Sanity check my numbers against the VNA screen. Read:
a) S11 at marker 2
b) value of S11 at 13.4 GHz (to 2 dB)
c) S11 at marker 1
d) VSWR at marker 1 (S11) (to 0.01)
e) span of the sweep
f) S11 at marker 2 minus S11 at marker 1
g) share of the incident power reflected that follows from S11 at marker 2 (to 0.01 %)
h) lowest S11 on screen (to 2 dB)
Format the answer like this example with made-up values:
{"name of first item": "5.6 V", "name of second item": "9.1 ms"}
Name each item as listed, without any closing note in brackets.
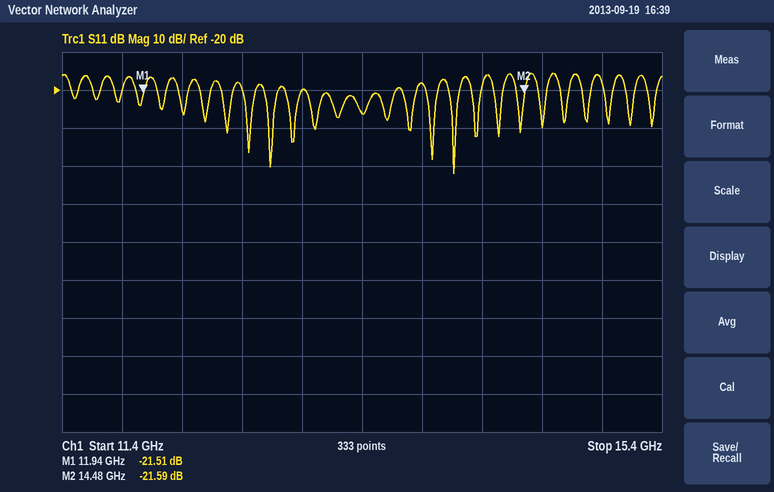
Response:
{"S11 at marker 2": "-21.59 dB", "value of S11 at 13.4 GHz": "-26 dB", "S11 at marker 1": "-21.51 dB", "VSWR at marker 1 (S11)": "1.18", "span of the sweep": "4 GHz", "S11 at marker 2 minus S11 at marker 1": "-0.08 dB", "share of the incident power reflected that follows from S11 at marker 2": "0.69 %", "lowest S11 on screen": "-42 dB"}
